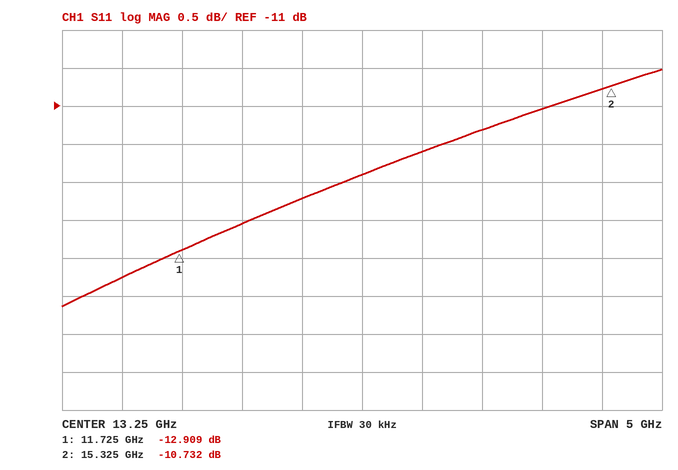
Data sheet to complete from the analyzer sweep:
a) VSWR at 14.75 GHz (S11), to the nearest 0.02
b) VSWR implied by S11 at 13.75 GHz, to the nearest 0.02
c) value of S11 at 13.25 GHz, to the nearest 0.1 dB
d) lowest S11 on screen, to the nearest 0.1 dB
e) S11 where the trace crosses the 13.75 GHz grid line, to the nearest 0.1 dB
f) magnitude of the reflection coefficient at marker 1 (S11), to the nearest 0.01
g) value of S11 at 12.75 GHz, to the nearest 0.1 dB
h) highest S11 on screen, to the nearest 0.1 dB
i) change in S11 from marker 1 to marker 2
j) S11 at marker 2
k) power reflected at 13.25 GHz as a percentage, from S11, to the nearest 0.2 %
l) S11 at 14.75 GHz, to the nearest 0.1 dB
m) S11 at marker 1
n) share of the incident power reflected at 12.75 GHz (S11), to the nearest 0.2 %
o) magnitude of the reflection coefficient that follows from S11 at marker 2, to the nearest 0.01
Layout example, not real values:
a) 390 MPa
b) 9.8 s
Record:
a) 1.78
b) 1.72
c) -11.9 dB
d) -13.6 dB
e) -11.6 dB
f) 0.23
g) -12.2 dB
h) -10.5 dB
i) 2.177 dB
j) -10.732 dB
k) 6.4 %
l) -11.0 dB
m) -12.909 dB
n) 6.0 %
o) 0.29
